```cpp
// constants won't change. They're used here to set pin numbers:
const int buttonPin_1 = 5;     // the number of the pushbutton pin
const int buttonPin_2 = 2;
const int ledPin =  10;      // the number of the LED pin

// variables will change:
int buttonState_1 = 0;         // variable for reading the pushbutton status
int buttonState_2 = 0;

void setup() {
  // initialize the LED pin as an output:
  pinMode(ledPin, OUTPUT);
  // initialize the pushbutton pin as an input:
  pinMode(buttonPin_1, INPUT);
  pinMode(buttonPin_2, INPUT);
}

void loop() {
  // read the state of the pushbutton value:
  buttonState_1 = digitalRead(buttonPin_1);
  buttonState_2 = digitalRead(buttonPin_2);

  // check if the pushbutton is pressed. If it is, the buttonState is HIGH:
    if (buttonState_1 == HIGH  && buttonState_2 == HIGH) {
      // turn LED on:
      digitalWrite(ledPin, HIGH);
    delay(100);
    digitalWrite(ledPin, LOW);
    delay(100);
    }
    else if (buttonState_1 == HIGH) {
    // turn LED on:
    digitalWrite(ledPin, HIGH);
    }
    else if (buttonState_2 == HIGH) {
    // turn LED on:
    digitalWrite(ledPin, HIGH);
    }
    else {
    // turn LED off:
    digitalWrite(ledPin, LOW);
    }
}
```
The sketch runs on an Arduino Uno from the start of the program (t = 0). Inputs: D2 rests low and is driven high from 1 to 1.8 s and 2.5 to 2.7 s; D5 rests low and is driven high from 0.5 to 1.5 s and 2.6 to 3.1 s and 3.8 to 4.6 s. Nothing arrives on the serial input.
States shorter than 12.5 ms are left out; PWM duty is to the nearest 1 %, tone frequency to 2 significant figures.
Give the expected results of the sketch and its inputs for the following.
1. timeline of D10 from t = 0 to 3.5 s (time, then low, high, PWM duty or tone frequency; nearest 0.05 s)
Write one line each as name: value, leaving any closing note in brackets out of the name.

timeline of D10 from t = 0 to 3.5 s: 0 s low; 0.5 s high; 1.1 s low; 1.2 s high; 1.3 s low; 1.4 s high; 1.5 s low; 1.6 s high; 1.8 s low; 2.5 s high; 2.7 s low; 2.8 s high; 3.1 s low
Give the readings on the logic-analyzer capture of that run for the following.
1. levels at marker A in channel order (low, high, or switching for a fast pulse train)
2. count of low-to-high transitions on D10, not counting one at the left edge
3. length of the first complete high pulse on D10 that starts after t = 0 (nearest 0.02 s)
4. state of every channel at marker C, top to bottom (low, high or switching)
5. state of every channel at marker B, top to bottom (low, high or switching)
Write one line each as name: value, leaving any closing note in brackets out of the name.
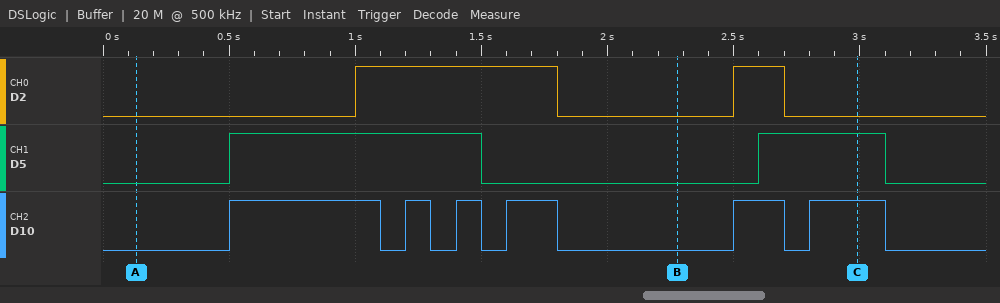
levels at marker A in channel order: D2 low, D5 low, D10 low
count of low-to-high transitions on D10, not counting one at the left edge: 6
length of the first complete high pulse on D10 that starts after t = 0: 0.60 s
state of every channel at marker C, top to bottom: D2 low, D5 high, D10 high
state of every channel at marker B, top to bottom: D2 low, D5 low, D10 low
